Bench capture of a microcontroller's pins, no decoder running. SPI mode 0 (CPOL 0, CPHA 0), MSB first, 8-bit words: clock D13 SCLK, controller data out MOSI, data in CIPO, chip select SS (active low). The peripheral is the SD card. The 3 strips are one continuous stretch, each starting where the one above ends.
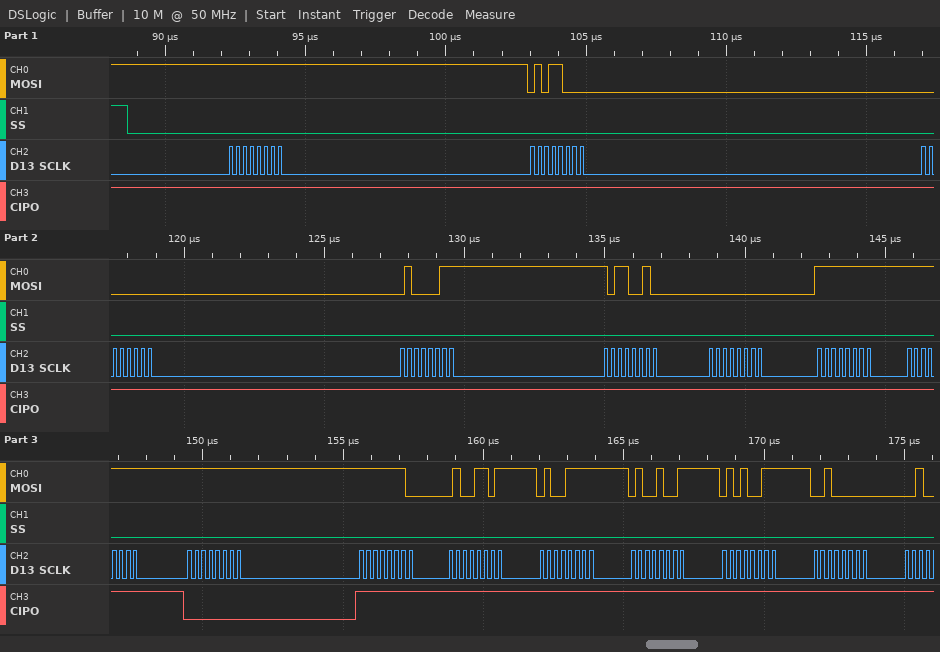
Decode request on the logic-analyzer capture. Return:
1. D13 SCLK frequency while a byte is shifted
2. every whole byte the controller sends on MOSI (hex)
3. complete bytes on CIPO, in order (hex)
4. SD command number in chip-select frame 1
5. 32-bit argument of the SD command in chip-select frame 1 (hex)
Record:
4 MHz
FF 58 00 43 B2 00 FF FF FF FE 4D 4F 49 53 20
FF FF FF FF FF FF FF FF 00 FF FF FF FF FF FF
CMD24
0x0043B200
